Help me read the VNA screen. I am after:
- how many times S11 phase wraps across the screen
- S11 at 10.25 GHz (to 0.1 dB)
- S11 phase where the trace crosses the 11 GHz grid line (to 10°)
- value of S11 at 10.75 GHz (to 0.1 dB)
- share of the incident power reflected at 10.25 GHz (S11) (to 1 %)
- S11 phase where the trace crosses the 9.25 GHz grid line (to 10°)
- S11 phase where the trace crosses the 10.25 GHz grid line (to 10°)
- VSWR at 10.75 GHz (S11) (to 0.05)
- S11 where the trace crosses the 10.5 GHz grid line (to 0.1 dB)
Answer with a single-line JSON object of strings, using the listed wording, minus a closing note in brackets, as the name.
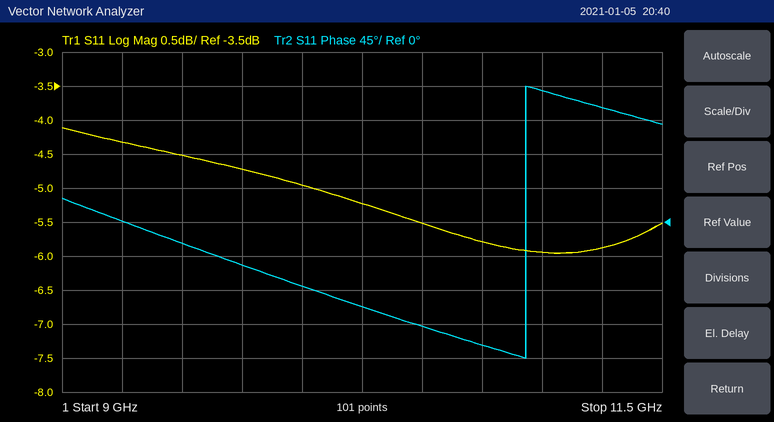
{"how many times S11 phase wraps across the screen": "1", "S11 at 10.25 GHz": "-5.2 dB", "S11 phase where the trace crosses the 11 GHz grid line": "170°", "value of S11 at 10.75 GHz": "-5.8 dB", "share of the incident power reflected at 10.25 GHz (S11)": "30 %", "S11 phase where the trace crosses the 9.25 GHz grid line": "0°", "S11 phase where the trace crosses the 10.25 GHz grid line": "-110°", "VSWR at 10.75 GHz (S11)": "3.10", "S11 where the trace crosses the 10.5 GHz grid line": "-5.5 dB"}
